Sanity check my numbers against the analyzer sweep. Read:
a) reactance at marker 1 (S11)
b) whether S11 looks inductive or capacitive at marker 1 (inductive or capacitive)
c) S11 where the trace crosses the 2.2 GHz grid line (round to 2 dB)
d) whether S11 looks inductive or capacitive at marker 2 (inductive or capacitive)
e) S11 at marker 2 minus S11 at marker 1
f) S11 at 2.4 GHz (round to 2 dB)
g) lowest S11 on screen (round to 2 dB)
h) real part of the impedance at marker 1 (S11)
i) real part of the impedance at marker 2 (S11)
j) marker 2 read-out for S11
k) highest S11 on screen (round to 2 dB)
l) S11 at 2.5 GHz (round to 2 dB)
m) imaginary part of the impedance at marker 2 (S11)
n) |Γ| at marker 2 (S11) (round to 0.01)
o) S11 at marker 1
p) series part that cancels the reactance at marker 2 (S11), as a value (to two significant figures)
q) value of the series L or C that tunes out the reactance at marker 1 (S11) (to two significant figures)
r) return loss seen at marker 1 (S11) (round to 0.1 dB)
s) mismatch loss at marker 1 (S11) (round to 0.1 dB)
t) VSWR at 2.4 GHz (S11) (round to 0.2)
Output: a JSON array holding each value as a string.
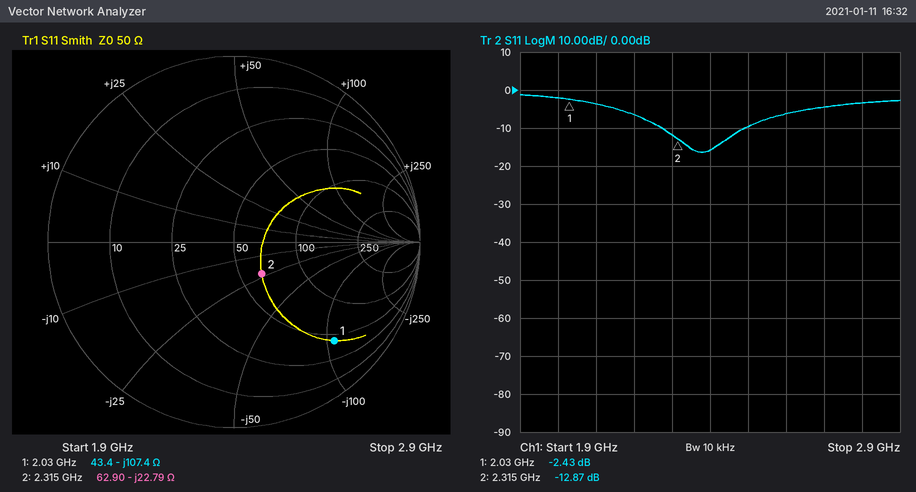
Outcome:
["-107.4 Ω", "capacitive", "-6 dB", "capacitive", "-10.44 dB", "-16 dB", "-16 dB", "43.4 Ω", "62.90 Ω", "-12.87 dB", "-2 dB", "-10 dB", "-22.79 Ω", "0.23", "-2.43 dB", "1.6 nH", "8.4 nH", "2.4 dB", "3.7 dB", "1.4"]
